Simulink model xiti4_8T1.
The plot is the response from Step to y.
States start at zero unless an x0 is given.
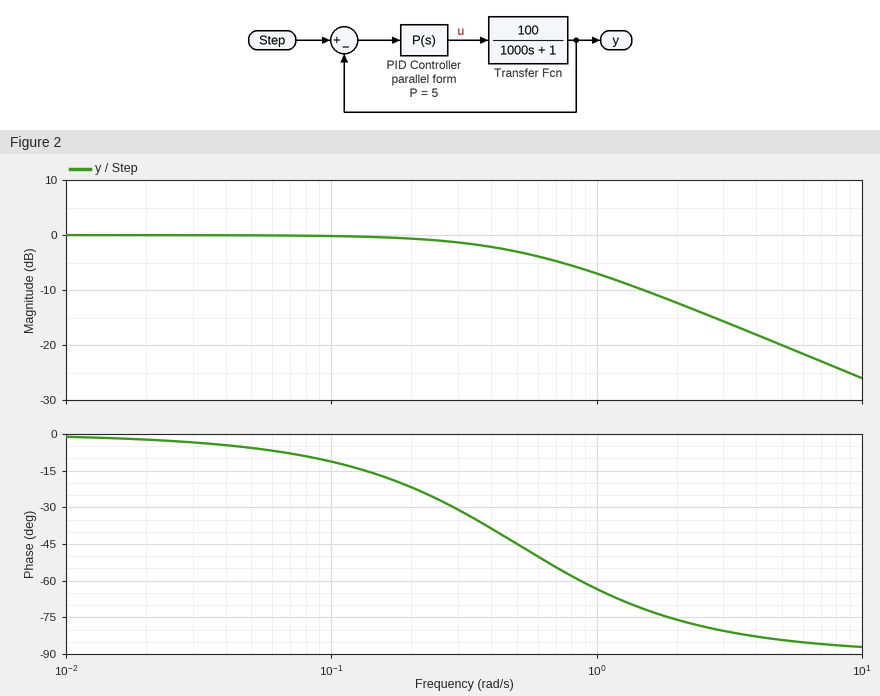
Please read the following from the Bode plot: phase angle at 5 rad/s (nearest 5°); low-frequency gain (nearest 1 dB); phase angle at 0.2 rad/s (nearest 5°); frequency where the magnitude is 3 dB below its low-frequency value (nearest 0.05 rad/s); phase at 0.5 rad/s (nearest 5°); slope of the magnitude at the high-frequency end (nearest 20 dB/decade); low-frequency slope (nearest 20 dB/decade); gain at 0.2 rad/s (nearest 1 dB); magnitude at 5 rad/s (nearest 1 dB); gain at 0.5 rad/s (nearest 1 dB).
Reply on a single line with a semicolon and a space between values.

-85°; 0 dB; -20°; 0.50 rad/s; -45°; -20 dB/decade; 0 dB/decade; -1 dB; -20 dB; -3 dB
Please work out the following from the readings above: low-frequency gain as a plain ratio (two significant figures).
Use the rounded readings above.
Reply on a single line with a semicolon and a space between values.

1.0
